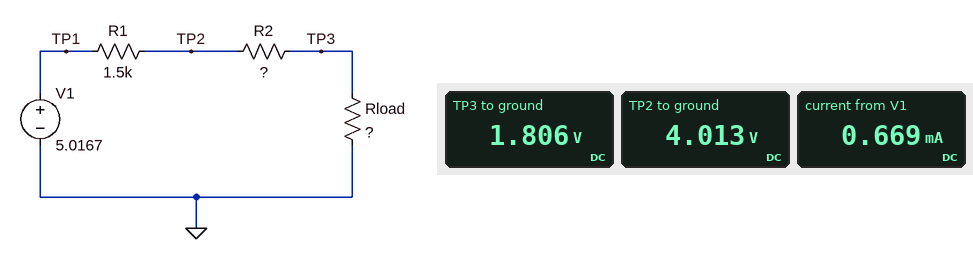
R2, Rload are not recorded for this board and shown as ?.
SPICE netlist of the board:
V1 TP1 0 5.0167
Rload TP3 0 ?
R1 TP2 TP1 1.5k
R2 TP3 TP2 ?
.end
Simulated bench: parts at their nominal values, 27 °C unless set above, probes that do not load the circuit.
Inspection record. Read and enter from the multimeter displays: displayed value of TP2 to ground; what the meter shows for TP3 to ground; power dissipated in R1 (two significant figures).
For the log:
4.013 V
1.806 V
670 µW
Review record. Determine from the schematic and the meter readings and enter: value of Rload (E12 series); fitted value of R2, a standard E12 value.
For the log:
2.7 kΩ
3.3 kΩ
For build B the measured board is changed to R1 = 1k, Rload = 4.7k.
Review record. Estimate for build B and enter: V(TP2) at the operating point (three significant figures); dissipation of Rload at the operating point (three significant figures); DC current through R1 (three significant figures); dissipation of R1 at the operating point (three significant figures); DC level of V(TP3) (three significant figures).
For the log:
4.46 V
1.46 mW
557 µA
311 µW
2.62 V
